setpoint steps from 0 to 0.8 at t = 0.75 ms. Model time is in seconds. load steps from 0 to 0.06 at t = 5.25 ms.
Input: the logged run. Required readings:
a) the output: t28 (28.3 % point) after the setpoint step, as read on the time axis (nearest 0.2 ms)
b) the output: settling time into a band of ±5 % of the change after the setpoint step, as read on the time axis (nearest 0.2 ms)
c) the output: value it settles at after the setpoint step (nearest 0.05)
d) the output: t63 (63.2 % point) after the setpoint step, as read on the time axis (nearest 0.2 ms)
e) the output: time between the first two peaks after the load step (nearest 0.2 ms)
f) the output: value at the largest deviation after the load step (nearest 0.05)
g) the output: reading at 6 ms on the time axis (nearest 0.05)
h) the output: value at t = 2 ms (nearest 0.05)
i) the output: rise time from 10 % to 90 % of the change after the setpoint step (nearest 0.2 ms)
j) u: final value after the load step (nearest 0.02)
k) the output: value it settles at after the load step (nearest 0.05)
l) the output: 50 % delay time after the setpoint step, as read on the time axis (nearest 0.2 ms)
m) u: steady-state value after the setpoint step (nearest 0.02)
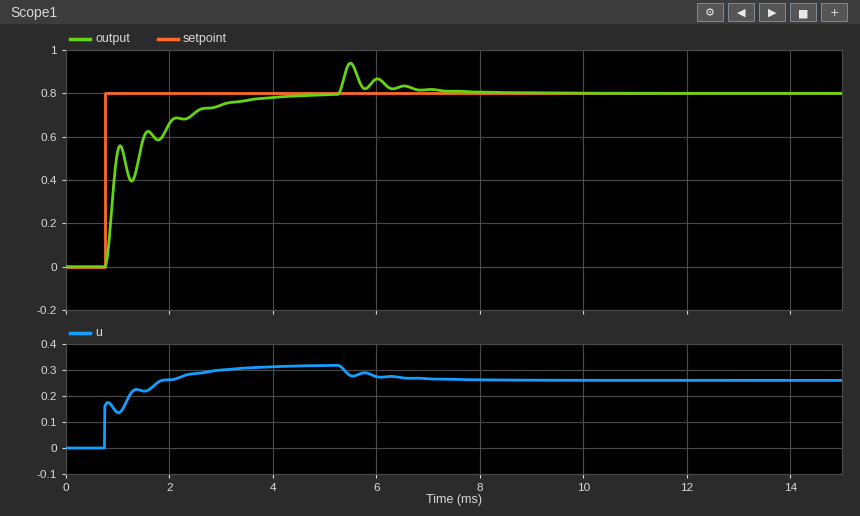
0.8 ms
3.2 ms
0.80
1.0 ms
0.6 ms
0.95
0.85
0.65
1.8 ms
0.26
0.80
1.0 ms
0.32
